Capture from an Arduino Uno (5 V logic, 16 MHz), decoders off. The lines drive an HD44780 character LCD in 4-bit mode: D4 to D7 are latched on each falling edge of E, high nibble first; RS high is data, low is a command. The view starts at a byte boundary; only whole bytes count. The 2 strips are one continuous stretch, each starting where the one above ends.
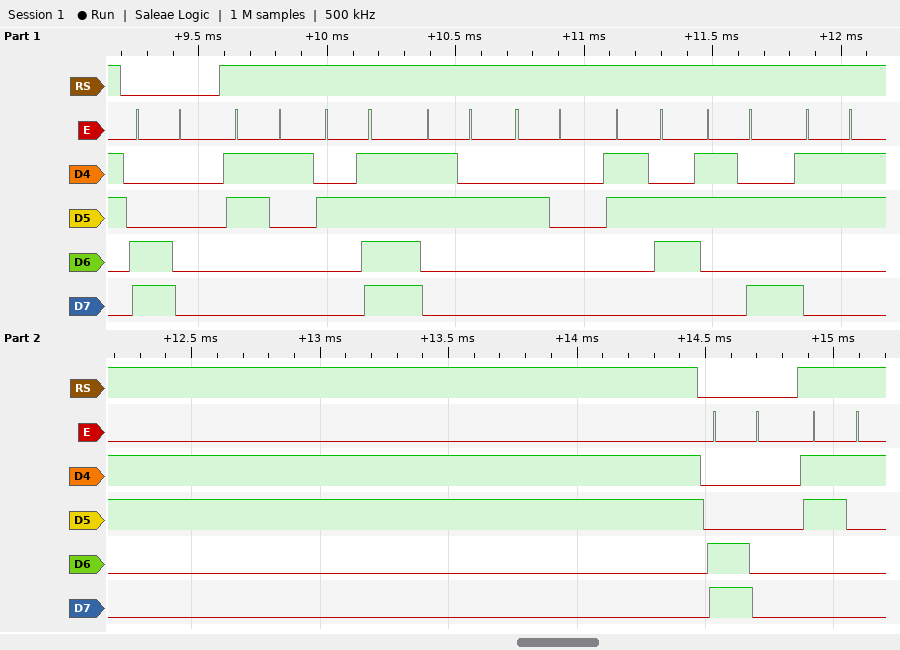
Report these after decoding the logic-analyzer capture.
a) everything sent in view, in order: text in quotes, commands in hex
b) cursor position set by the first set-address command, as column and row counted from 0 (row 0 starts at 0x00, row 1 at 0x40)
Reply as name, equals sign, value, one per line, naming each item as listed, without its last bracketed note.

everything sent in view, in order: text in quotes, commands in hex = 0xC0 "1/2 6:3" 0xC0 "1"
cursor position set by the first set-address command, as column and row counted from 0 = column 0, row 1
